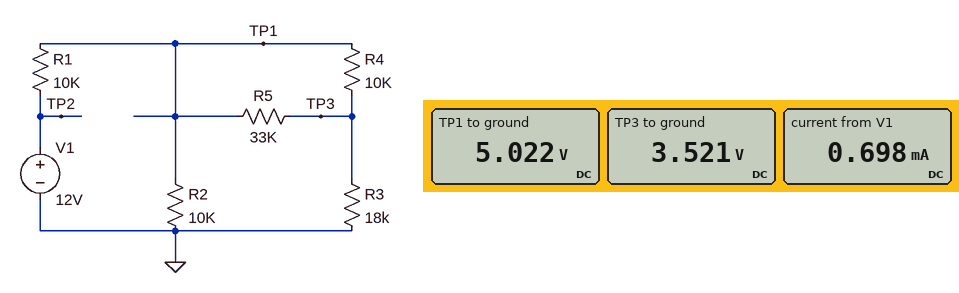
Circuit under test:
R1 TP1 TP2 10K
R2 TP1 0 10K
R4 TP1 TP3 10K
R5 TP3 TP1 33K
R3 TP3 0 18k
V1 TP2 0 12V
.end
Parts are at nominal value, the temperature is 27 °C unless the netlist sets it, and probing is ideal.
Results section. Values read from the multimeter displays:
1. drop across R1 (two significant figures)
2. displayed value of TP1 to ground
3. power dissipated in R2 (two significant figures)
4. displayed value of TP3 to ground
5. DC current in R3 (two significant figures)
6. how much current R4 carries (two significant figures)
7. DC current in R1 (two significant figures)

7.0 V
5.022 V
2.5 mW
3.521 V
200 µA
150 µA
700 µA
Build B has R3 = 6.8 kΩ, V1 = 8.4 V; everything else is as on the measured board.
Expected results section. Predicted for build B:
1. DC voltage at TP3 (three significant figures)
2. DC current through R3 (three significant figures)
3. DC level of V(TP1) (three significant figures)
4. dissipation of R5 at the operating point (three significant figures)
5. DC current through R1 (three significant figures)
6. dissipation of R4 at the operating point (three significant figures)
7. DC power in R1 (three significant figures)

1.47 V
216 µA
3.12 V
83.0 µW
528 µA
274 µW
2.79 mW
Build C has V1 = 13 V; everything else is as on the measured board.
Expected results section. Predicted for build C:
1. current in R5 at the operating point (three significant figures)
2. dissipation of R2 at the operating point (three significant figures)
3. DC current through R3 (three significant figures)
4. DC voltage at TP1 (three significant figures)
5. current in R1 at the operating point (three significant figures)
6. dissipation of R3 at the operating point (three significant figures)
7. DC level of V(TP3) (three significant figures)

49.3 µA
2.96 mW
212 µA
5.44 V
756 µA
808 µW
3.81 V
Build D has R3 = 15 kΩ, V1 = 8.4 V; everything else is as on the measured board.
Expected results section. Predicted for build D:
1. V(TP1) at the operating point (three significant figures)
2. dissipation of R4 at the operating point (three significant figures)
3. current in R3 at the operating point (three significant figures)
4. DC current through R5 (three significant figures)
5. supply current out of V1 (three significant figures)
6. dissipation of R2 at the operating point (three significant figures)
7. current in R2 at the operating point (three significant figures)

3.44 V
136 µW
152 µA
35.3 µA
496 µA
1.18 mW
344 µA
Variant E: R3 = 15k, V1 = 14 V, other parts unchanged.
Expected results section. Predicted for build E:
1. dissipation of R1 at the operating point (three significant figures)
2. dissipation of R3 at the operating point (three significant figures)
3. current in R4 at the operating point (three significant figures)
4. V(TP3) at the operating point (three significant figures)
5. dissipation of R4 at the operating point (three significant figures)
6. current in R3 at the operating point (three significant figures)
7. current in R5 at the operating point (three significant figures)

6.83 mW
960 µW
194 µA
3.79 V
377 µW
253 µA
58.8 µA
